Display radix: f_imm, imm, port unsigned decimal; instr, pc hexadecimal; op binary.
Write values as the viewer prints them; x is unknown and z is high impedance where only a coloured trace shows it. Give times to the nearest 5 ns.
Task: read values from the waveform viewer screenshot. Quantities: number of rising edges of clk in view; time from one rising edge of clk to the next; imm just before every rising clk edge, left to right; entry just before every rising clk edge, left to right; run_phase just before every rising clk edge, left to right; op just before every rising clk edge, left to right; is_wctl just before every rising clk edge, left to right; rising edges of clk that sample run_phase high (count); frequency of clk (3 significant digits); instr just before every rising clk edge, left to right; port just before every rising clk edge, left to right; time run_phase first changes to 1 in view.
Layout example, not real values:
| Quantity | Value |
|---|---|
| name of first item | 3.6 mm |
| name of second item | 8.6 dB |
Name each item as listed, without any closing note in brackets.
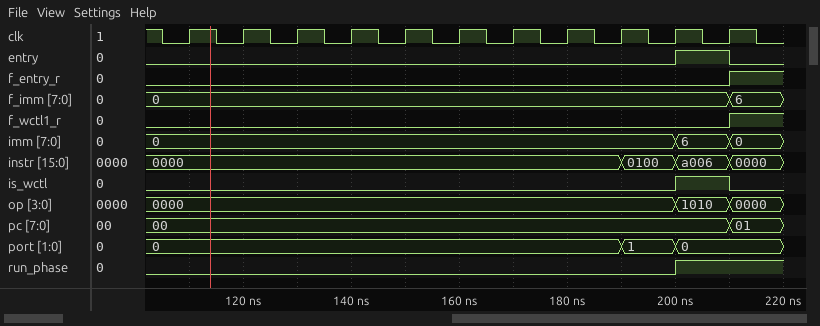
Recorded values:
| Quantity | Value |
|---|---|
| number of rising edges of clk in view | 11 |
| time from one rising edge of clk to the next | 10 ns |
| imm just before every rising clk edge, left to right | 0, 0, 0, 0, 0, 0, 0, 0, 0, 0, 6 |
| entry just before every rising clk edge, left to right | 0 0 0 0 0 0 0 0 0 0 1 |
| run_phase just before every rising clk edge, left to right | 0 0 0 0 0 0 0 0 0 0 1 |
| op just before every rising clk edge, left to right | 0000, 0000, 0000, 0000, 0000, 0000, 0000, 0000, 0000, 0000, 1010 |
| is_wctl just before every rising clk edge, left to right | 0 0 0 0 0 0 0 0 0 0 1 |
| rising edges of clk that sample run_phase high | 1 |
| frequency of clk | 100 MHz |
| instr just before every rising clk edge, left to right | 0000, 0000, 0000, 0000, 0000, 0000, 0000, 0000, 0000, 0100, a006 |
| port just before every rising clk edge, left to right | 0, 0, 0, 0, 0, 0, 0, 0, 0, 1, 0 |
| time run_phase first changes to 1 in view | 200 ns |
